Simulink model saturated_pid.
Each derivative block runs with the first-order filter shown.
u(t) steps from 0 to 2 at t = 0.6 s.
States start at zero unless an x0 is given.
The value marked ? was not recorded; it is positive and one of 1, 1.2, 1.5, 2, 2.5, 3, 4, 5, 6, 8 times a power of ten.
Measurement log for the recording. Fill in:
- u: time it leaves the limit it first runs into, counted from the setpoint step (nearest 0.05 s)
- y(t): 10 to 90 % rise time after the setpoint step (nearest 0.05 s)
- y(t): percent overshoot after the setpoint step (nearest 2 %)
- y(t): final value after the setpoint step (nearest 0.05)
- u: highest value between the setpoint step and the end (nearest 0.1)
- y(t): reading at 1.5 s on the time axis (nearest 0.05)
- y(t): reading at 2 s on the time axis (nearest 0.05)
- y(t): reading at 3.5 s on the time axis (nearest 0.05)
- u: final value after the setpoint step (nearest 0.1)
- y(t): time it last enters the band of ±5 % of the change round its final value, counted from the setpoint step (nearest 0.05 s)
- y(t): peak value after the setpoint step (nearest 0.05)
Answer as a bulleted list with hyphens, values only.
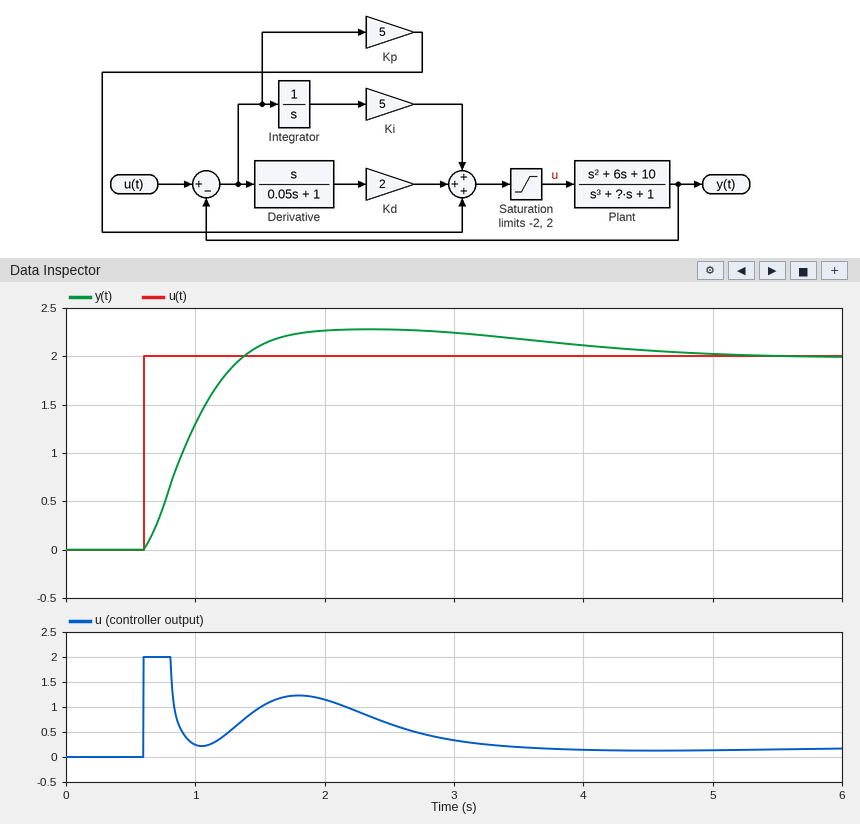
- 0.20 s
- 0.55 s
- 14 %
- 2.00
- 2.0
- 2.10
- 2.25
- 2.20
- 0.2
- 3.50 s
- 2.30
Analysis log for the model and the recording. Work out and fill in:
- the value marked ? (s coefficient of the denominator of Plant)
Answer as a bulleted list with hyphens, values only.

- 8
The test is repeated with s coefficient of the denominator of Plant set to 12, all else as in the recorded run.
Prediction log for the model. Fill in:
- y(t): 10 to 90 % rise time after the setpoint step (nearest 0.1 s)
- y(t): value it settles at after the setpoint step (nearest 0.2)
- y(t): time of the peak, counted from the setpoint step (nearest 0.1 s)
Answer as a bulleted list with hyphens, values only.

- 0.6 s
- 2.0
- 2.1 s
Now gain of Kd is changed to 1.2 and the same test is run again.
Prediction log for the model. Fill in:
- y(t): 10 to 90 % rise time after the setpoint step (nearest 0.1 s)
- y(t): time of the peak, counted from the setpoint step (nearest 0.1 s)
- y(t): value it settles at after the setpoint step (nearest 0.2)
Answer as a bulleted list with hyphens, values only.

- 0.4 s
- 0.9 s
- 2.0
